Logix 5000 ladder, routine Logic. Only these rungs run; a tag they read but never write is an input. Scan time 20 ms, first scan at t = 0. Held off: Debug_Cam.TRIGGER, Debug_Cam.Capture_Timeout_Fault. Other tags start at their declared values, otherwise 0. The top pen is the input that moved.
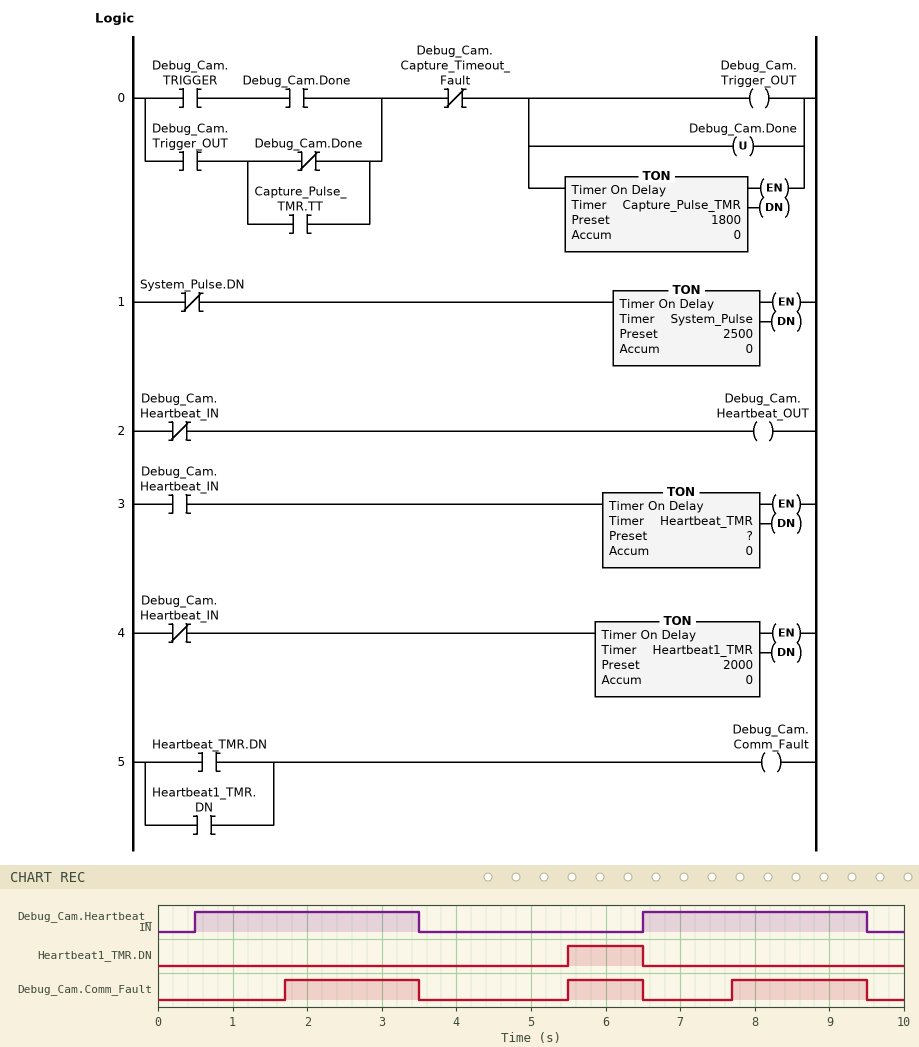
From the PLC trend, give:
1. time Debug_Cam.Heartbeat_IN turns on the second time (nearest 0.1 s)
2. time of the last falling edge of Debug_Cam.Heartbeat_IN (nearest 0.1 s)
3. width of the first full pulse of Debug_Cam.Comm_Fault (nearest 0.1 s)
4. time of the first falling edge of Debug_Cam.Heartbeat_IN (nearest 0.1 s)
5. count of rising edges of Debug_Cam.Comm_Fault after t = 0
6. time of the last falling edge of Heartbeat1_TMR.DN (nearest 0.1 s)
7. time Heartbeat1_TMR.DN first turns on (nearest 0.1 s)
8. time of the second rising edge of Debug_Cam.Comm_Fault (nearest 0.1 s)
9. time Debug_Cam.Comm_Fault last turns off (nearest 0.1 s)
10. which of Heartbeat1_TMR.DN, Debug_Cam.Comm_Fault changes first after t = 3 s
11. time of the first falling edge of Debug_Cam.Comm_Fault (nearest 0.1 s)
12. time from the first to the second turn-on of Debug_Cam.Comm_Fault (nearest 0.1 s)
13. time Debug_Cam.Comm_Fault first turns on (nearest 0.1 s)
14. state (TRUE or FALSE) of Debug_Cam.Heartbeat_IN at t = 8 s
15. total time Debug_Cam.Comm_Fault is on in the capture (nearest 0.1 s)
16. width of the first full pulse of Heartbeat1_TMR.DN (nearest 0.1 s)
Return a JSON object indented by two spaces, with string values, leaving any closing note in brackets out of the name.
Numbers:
{
  "time Debug_Cam.Heartbeat_IN turns on the second time": "6.5 s",
  "time of the last falling edge of Debug_Cam.Heartbeat_IN": "9.5 s",
  "width of the first full pulse of Debug_Cam.Comm_Fault": "1.8 s",
  "time of the first falling edge of Debug_Cam.Heartbeat_IN": "3.5 s",
  "count of rising edges of Debug_Cam.Comm_Fault after t = 0": "3",
  "time of the last falling edge of Heartbeat1_TMR.DN": "6.5 s",
  "time Heartbeat1_TMR.DN first turns on": "5.5 s",
  "time of the second rising edge of Debug_Cam.Comm_Fault": "5.5 s",
  "time Debug_Cam.Comm_Fault last turns off": "9.5 s",
  "which of Heartbeat1_TMR.DN, Debug_Cam.Comm_Fault changes first after t = 3 s": "Debug_Cam.Comm_Fault",
  "time of the first falling edge of Debug_Cam.Comm_Fault": "3.5 s",
  "time from the first to the second turn-on of Debug_Cam.Comm_Fault": "3.8 s",
  "time Debug_Cam.Comm_Fault first turns on": "1.7 s",
  "state (TRUE or FALSE) of Debug_Cam.Heartbeat_IN at t = 8 s": "TRUE",
  "total time Debug_Cam.Comm_Fault is on in the capture": "4.6 s",
  "width of the first full pulse of Heartbeat1_TMR.DN": "1.0 s"
}
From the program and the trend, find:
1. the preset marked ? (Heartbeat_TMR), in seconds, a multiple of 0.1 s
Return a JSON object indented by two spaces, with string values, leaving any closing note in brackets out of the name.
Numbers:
{
  "the preset marked ? (Heartbeat_TMR), in seconds, a multiple of 0.1 s": "1.2 s"
}
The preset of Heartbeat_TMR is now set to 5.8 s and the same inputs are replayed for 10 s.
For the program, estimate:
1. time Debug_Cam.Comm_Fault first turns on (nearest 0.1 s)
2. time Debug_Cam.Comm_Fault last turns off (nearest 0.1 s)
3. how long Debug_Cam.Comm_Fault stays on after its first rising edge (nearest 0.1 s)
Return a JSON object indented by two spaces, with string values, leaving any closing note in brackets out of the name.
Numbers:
{
  "time Debug_Cam.Comm_Fault first turns on": "5.5 s",
  "time Debug_Cam.Comm_Fault last turns off": "6.5 s",
  "how long Debug_Cam.Comm_Fault stays on after its first rising edge": "1.0 s"
}
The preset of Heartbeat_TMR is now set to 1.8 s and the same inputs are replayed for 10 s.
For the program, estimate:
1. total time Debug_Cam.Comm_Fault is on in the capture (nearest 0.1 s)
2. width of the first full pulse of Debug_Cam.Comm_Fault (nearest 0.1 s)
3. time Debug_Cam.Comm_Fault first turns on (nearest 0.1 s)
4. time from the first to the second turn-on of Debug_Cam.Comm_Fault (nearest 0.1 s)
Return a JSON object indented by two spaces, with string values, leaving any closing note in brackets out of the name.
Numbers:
{
  "total time Debug_Cam.Comm_Fault is on in the capture": "3.4 s",
  "width of the first full pulse of Debug_Cam.Comm_Fault": "1.2 s",
  "time Debug_Cam.Comm_Fault first turns on": "2.3 s",
  "time from the first to the second turn-on of Debug_Cam.Comm_Fault": "3.2 s"
}
